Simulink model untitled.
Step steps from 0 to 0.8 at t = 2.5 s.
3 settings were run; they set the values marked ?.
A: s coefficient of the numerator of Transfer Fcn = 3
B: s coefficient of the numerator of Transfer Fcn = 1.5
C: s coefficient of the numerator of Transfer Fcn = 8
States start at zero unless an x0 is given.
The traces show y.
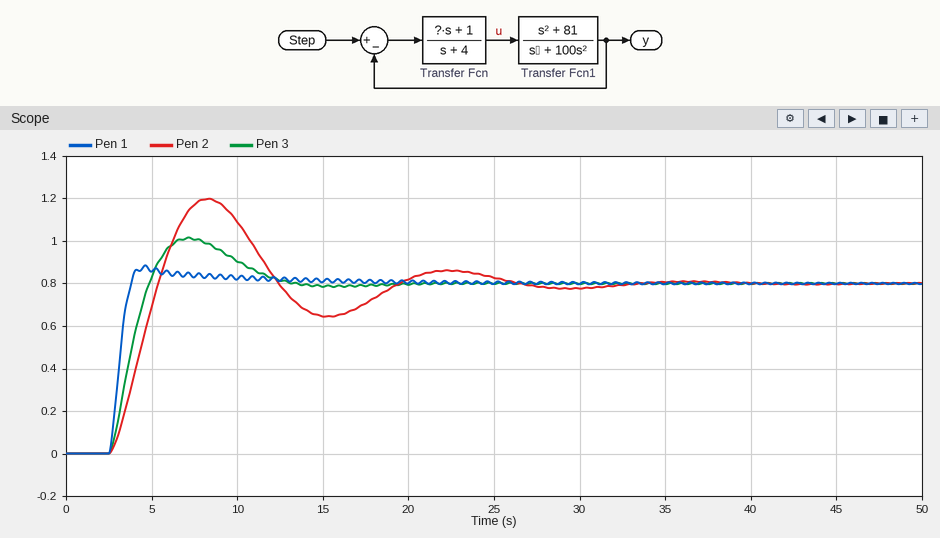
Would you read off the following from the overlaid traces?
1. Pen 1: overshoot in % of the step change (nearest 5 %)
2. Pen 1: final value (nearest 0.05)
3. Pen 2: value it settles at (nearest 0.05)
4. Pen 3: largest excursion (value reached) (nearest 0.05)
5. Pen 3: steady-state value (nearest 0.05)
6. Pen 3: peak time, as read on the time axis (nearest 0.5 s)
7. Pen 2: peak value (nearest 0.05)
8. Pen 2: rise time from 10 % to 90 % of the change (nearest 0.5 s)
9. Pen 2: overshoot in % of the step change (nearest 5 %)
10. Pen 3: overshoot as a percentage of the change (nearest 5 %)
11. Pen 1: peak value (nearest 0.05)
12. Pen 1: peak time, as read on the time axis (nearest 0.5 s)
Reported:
10 %
0.80
0.80
1.00
0.80
7.0 s
1.20
2.0 s
50 %
25 %
0.90
4.5 s
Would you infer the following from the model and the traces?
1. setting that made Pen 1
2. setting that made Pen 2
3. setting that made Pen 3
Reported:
C
B
A
